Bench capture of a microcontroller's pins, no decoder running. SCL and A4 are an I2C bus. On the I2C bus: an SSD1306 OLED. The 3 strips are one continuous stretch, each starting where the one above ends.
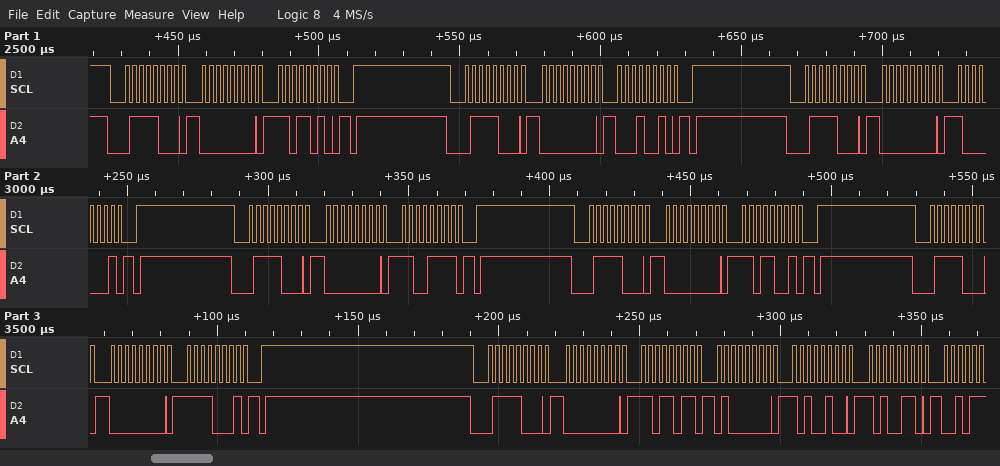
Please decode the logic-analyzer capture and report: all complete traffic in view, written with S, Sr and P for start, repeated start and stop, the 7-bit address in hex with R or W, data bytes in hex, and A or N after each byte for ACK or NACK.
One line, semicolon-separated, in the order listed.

S 3CW A 00 A DA A P S 3CW A 00 A 12 A P S 3CW A 00 A 81 A P S 3CW A 00 A CF A P S 3CW A 00 A D9 A P S 3CW A 00 A F1 A P S 3CW A 00 A DB A 40 A A4 A A6 A
